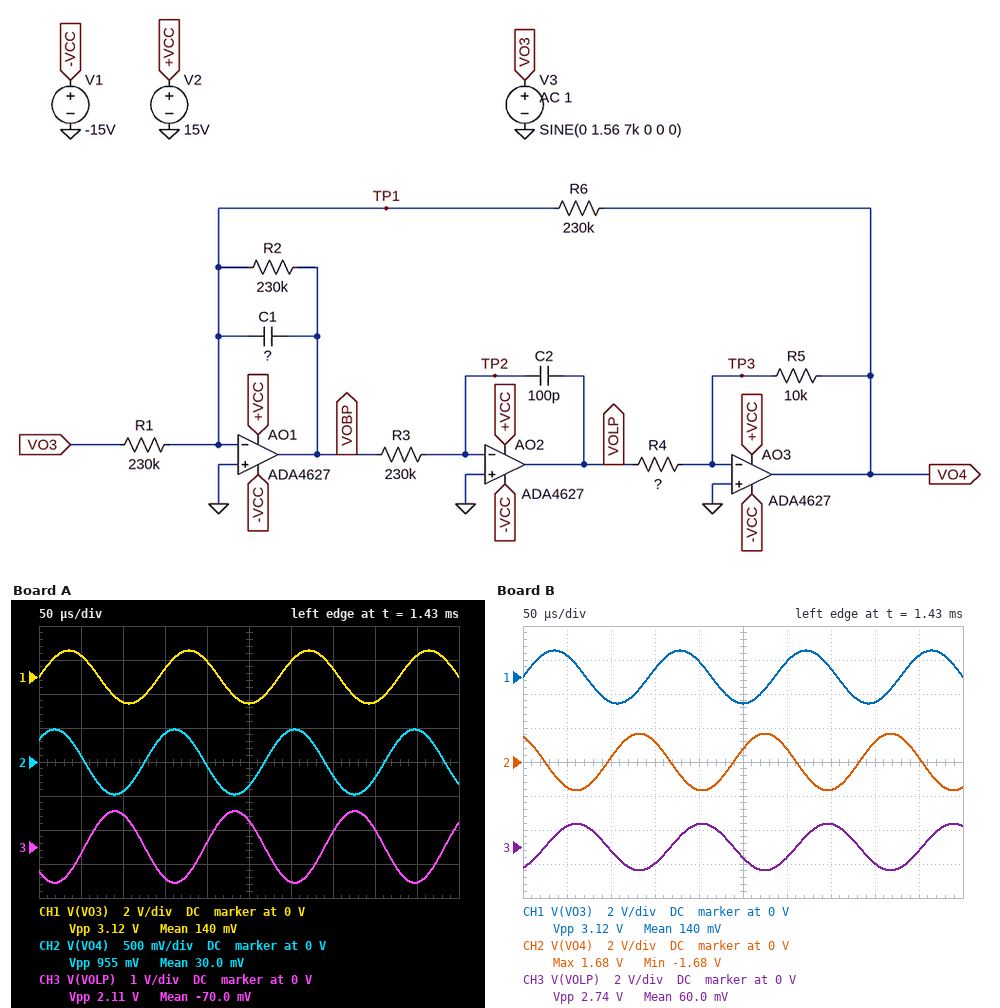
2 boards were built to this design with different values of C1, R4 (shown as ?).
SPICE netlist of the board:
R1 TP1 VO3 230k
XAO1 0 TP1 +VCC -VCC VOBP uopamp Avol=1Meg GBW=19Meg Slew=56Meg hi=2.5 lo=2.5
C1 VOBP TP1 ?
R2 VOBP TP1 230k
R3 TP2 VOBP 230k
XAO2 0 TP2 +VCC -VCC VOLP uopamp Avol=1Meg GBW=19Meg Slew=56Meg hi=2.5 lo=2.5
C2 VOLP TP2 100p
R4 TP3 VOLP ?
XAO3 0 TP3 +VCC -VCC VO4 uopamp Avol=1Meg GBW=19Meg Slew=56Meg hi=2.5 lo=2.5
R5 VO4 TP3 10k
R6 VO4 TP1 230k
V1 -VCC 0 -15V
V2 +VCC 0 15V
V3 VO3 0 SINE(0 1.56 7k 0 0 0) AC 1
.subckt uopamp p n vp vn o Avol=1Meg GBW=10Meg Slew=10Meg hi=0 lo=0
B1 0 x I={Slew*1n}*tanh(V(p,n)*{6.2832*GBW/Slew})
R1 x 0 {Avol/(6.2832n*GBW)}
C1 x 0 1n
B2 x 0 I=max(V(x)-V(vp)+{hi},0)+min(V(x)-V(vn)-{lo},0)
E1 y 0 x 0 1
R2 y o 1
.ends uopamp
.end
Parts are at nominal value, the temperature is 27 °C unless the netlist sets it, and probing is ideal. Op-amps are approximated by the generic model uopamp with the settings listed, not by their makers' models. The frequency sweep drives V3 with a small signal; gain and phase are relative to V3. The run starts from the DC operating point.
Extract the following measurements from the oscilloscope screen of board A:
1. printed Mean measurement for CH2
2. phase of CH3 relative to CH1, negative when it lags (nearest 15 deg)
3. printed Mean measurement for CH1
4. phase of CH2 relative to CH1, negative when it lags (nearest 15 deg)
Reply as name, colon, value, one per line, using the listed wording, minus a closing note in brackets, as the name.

printed Mean measurement for CH2: 30.0 mV
phase of CH3 relative to CH1, negative when it lags: -135 deg
printed Mean measurement for CH1: 140 mV
phase of CH2 relative to CH1, negative when it lags: 45 deg
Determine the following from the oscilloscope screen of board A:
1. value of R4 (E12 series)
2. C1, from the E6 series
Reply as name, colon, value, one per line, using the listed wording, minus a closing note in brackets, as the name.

value of R4: 22 kΩ
C1, from the E6 series: 150 pF
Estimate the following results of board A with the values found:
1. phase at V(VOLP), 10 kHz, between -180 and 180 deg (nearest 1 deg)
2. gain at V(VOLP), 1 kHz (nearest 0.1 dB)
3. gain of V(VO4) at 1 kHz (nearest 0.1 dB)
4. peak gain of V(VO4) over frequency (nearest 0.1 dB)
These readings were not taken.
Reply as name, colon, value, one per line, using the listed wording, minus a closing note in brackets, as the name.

phase at V(VOLP), 10 kHz, between -180 and 180 deg: -152 deg
gain at V(VOLP), 1 kHz: 7.0 dB
gain of V(VO4) at 1 kHz: 0.1 dB
peak gain of V(VO4) over frequency: 0.3 dB
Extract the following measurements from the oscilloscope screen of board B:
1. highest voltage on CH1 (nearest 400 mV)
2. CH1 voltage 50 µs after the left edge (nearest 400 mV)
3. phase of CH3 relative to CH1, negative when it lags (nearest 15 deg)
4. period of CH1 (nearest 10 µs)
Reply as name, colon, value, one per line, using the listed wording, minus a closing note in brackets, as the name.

highest voltage on CH1: 1.6 V
CH1 voltage 50 µs after the left edge: 1.2 V
phase of CH3 relative to CH1, negative when it lags: -60 deg
period of CH1: 140 µs
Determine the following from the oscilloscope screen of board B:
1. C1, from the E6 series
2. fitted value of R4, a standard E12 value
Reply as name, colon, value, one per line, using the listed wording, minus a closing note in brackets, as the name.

C1, from the E6 series: 68 pF
fitted value of R4, a standard E12 value: 8.2 kΩ
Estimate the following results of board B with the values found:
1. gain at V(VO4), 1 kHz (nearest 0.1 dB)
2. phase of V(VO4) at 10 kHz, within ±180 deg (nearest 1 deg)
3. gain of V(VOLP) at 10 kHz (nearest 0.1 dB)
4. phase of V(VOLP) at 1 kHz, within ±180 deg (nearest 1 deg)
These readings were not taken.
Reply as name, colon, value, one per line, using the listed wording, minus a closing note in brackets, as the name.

gain at V(VO4), 1 kHz: 0 dB
phase of V(VO4) at 10 kHz, within ±180 deg: 82 deg
gain of V(VOLP) at 10 kHz: -3.3 dB
phase of V(VOLP) at 1 kHz, within ±180 deg: -7 deg
